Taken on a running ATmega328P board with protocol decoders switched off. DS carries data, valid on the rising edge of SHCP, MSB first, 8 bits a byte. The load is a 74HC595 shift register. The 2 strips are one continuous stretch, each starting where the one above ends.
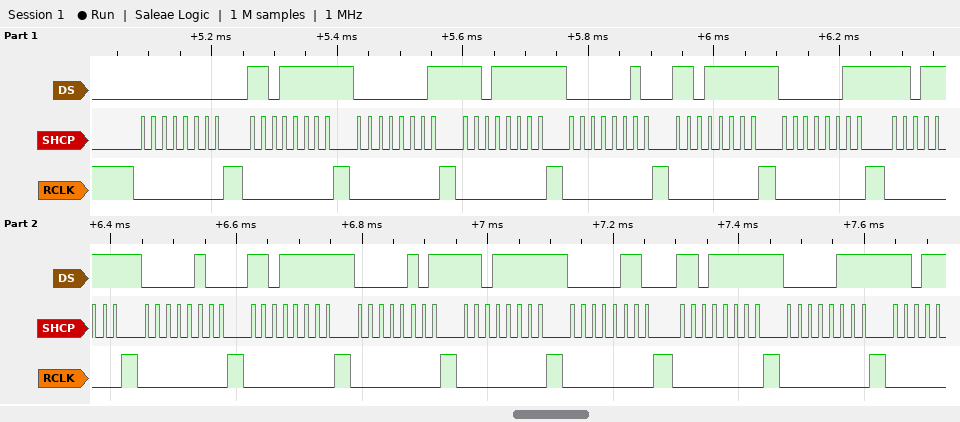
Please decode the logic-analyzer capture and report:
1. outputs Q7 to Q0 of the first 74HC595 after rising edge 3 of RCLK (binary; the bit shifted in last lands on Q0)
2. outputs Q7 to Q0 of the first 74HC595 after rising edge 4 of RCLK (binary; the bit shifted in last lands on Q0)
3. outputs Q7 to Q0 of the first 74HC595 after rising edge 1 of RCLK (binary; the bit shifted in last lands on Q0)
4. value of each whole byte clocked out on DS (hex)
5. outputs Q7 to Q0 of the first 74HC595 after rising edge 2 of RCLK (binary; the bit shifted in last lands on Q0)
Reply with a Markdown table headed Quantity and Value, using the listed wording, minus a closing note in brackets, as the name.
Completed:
| Quantity | Value |
|---|---|
| outputs Q7 to Q0 of the first 74HC595 after rising edge 3 of RCLK | 00000001 |
| outputs Q7 to Q0 of the first 74HC595 after rising edge 4 of RCLK | 11011111 |
| outputs Q7 to Q0 of the first 74HC595 after rising edge 1 of RCLK | 00000000 |
| value of each whole byte clocked out on DS | 00 DF 01 DF 02 DF 03 DF 04 DF 05 DF 06 DF 07 |
| outputs Q7 to Q0 of the first 74HC595 after rising edge 2 of RCLK | 11011111 |
